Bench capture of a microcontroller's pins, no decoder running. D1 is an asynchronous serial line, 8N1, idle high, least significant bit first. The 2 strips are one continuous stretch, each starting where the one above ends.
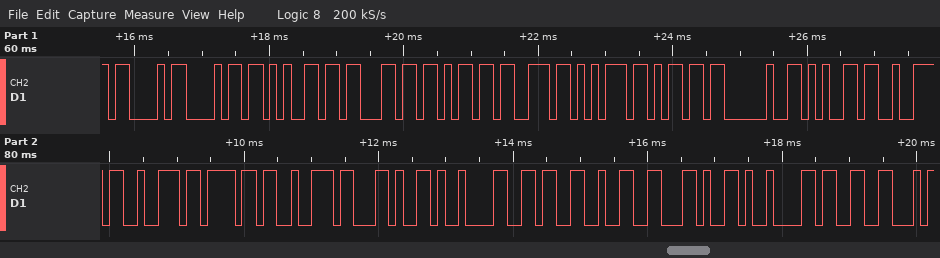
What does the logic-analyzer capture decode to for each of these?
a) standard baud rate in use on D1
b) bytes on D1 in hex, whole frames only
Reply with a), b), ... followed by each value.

a) 9600 baud
b) 43 68 65 63 6B 73 75 6D 20 65 72 72 6F 72 2C 09 36 32 2C 09 33
